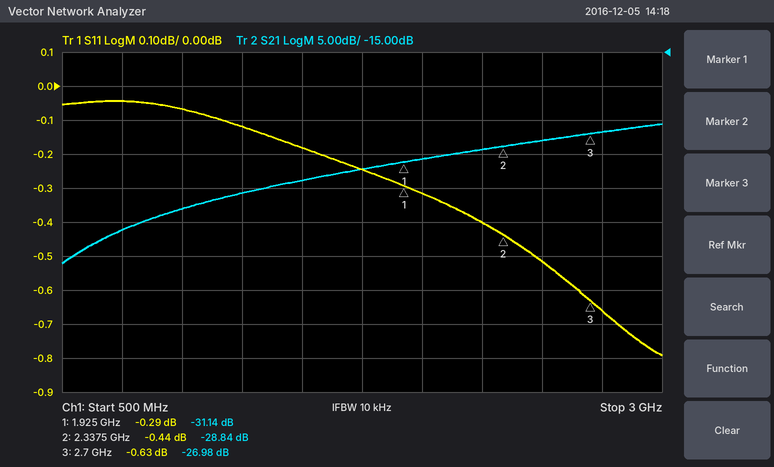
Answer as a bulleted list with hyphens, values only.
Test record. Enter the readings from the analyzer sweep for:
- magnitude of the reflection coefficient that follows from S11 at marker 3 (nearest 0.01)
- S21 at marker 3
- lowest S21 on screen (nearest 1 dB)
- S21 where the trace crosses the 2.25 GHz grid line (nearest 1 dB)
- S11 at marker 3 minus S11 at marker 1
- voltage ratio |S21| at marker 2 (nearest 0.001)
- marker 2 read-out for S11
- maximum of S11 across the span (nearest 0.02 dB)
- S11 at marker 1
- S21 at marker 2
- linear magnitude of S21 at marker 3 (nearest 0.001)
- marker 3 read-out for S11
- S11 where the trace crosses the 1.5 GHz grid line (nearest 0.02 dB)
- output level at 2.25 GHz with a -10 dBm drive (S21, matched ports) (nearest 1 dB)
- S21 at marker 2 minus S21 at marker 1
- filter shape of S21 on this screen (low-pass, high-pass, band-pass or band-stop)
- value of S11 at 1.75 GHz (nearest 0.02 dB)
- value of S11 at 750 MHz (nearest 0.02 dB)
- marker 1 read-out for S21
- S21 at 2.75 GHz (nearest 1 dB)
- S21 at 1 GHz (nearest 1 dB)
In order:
- 0.93
- -26.98 dB
- -46 dB
- -29 dB
- -0.34 dB
- 0.036
- -0.44 dB
- -0.04 dB
- -0.29 dB
- -28.84 dB
- 0.045
- -0.63 dB
- -0.18 dB
- -39 dBm
- 2.30 dB
- high-pass
- -0.24 dB
- -0.04 dB
- -31.14 dB
- -27 dB
- -38 dB
